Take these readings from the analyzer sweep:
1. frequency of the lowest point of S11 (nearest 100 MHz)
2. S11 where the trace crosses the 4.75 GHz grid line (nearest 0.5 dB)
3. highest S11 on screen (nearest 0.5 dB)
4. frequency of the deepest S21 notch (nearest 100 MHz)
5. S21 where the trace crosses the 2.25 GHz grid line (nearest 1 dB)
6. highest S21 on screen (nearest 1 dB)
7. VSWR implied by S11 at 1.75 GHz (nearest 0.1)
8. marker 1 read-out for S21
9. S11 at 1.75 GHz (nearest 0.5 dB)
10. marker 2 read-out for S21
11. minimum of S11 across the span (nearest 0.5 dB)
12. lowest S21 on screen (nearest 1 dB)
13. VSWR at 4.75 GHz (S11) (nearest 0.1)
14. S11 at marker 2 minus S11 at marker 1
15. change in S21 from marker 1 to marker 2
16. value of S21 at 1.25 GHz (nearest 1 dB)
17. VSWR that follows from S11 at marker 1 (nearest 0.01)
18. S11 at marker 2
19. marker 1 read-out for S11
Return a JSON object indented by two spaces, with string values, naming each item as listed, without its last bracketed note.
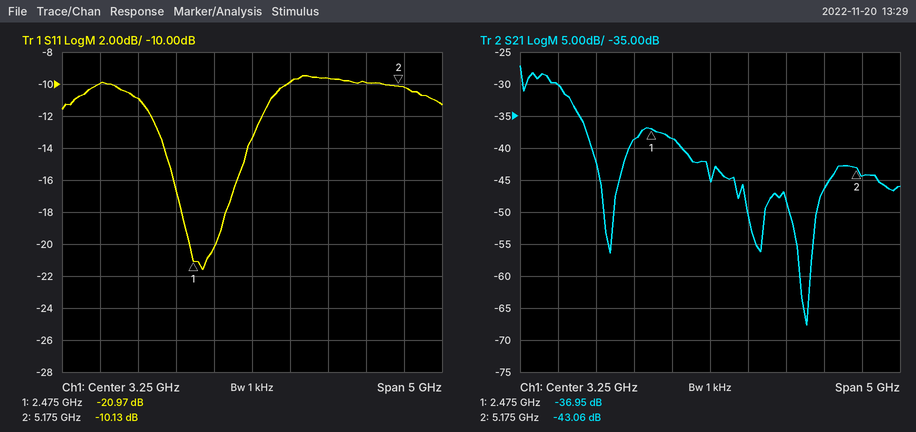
{
  "frequency of the lowest point of S11": "2.6 GHz",
  "S11 where the trace crosses the 4.75 GHz grid line": "-10.0 dB",
  "highest S11 on screen": "-9.5 dB",
  "frequency of the deepest S21 notch": "4.5 GHz",
  "S21 where the trace crosses the 2.25 GHz grid line": "-39 dB",
  "highest S21 on screen": "-27 dB",
  "VSWR implied by S11 at 1.75 GHz": "1.8",
  "marker 1 read-out for S21": "-36.95 dB",
  "S11 at 1.75 GHz": "-11.0 dB",
  "marker 2 read-out for S21": "-43.06 dB",
  "minimum of S11 across the span": "-21.5 dB",
  "lowest S21 on screen": "-68 dB",
  "VSWR at 4.75 GHz (S11)": "1.9",
  "S11 at marker 2 minus S11 at marker 1": "10.84 dB",
  "change in S21 from marker 1 to marker 2": "-6.11 dB",
  "value of S21 at 1.25 GHz": "-30 dB",
  "VSWR that follows from S11 at marker 1": "1.20",
  "S11 at marker 2": "-10.13 dB",
  "marker 1 read-out for S11": "-20.97 dB"
}
